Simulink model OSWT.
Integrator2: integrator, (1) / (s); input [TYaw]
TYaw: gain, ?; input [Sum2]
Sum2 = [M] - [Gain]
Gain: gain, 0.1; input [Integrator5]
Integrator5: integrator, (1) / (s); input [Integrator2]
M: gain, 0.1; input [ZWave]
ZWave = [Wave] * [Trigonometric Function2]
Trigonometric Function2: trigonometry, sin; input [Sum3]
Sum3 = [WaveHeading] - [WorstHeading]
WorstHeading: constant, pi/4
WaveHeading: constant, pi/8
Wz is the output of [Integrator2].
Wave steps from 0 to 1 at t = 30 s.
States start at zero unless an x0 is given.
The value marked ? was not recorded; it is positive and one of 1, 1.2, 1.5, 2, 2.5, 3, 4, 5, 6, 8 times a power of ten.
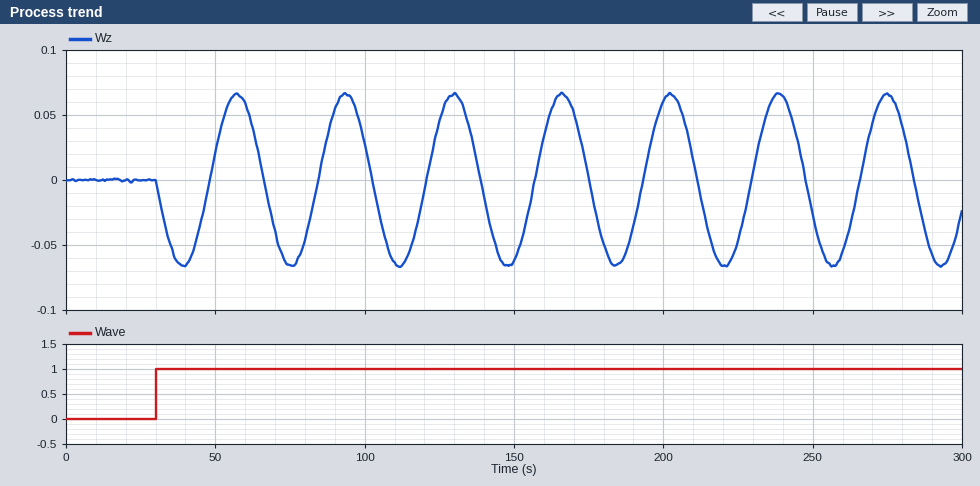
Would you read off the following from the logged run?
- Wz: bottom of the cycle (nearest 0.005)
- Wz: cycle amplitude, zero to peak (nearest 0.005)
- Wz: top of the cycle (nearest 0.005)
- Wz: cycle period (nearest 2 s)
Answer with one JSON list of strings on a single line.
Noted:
["-0.065", "0.065", "0.065", "36 s"]
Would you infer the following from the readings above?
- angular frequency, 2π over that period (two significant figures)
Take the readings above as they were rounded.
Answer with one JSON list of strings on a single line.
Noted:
["0.17 rad/s"]
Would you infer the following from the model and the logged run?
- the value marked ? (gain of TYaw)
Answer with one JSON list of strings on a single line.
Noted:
["0.3"]
